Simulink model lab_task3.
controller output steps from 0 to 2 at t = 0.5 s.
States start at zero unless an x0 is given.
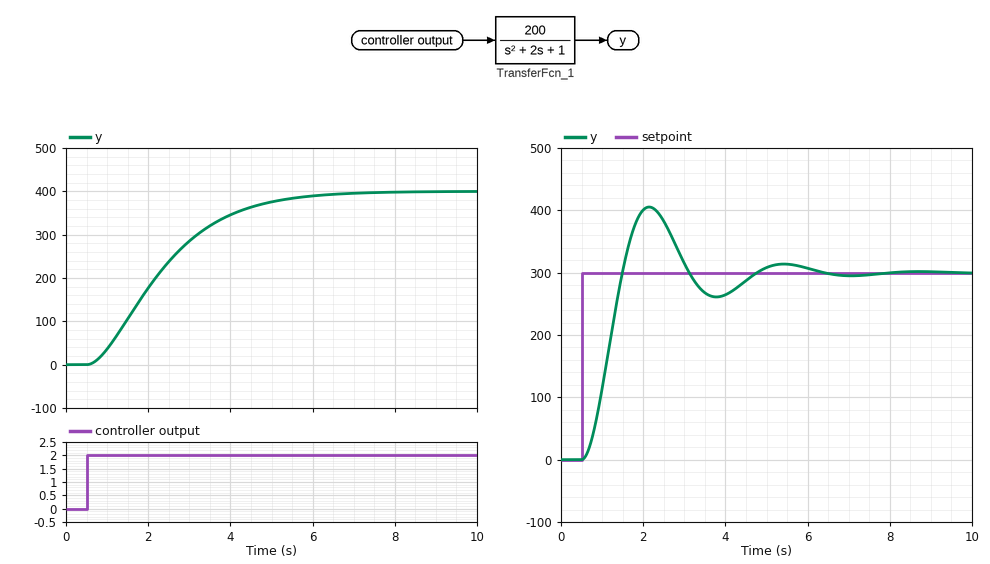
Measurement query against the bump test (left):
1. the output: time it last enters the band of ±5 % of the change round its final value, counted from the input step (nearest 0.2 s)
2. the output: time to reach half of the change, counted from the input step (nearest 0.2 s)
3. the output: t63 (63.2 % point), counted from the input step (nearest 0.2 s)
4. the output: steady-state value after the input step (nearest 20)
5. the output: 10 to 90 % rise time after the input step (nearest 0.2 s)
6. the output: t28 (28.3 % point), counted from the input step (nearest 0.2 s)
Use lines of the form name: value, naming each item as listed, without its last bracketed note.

the output: time it last enters the band of ±5 % of the change round its final value, counted from the input step: 4.8 s
the output: time to reach half of the change, counted from the input step: 1.6 s
the output: t63 (63.2 % point), counted from the input step: 2.2 s
the output: steady-state value after the input step: 400
the output: 10 to 90 % rise time after the input step: 3.4 s
the output: t28 (28.3 % point), counted from the input step: 1.0 s
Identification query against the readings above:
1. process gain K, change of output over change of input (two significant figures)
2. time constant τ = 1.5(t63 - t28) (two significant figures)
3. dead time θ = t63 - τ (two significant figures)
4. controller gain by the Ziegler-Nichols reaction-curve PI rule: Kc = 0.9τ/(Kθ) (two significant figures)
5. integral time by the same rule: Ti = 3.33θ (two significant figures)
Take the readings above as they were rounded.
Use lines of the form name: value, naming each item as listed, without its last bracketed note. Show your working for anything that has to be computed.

process gain K, change of output over change of input: (400 - 0) / 2 = 200
time constant τ = 1.5(t63 - t28): 1.5 × (2.2 - 1) = 1.8 s
dead time θ = t63 - τ: 2.2 - 1.8 = 0.40 s
controller gain by the Ziegler-Nichols reaction-curve PI rule: Kc = 0.9τ/(Kθ): 0.9 × 1.8 / (200 × 0.4) = 0.020
integral time by the same rule: Ti = 3.33θ: 3.33 × 0.4 = 1.3 s
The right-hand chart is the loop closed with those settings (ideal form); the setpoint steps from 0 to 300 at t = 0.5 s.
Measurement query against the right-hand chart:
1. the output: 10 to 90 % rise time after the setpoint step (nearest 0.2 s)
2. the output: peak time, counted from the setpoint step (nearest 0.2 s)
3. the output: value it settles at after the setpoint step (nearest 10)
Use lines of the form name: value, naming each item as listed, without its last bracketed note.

the output: 10 to 90 % rise time after the setpoint step: 0.6 s
the output: peak time, counted from the setpoint step: 1.6 s
the output: value it settles at after the setpoint step: 300
